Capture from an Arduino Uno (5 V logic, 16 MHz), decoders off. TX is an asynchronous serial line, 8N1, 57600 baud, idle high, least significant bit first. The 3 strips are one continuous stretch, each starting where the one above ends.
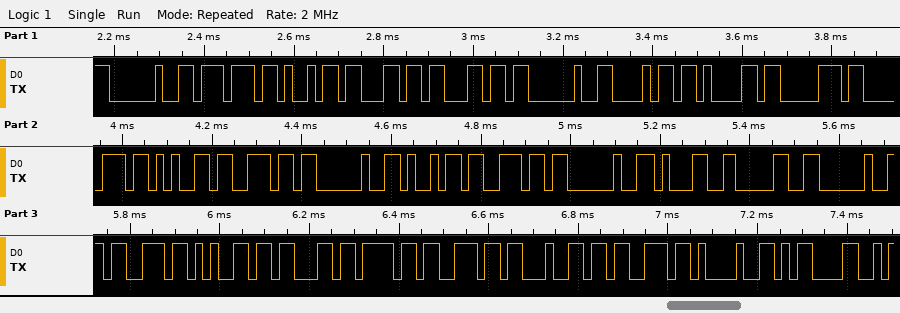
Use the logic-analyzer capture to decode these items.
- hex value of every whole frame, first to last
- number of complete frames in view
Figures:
0x20 0x77 0x69 0x6C 0x6C 0x20 0x68 0x61 0x70 0x70 0x65 0x6E 0x20 0x69 0x6E 0x20 0x31 0x30 0x20 0x73 0x65 0x63 0x6F 0x6E 0x64 0x73 0x21 0x0D
28
